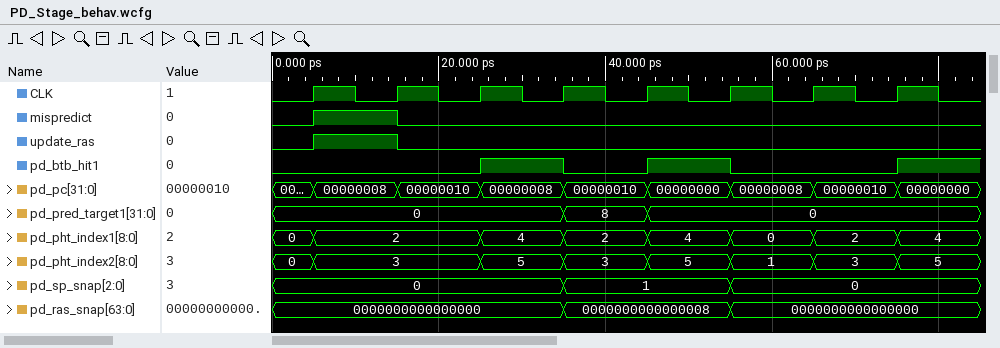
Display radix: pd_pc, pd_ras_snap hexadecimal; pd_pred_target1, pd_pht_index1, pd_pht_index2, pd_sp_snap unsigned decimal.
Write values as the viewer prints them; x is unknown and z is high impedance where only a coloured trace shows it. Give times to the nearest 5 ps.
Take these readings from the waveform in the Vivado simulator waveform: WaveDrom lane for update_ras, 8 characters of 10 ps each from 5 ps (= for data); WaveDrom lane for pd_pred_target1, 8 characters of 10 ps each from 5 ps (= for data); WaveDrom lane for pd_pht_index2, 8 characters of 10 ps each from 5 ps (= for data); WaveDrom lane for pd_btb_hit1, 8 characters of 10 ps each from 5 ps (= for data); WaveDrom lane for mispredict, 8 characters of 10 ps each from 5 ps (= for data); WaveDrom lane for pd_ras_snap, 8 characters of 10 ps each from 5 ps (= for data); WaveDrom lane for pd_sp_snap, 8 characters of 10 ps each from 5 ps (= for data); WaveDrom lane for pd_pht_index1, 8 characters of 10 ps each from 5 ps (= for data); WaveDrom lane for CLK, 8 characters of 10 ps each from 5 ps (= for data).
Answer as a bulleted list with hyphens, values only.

- {name: 'update_ras', wave: '10......'}
- {name: 'pd_pred_target1', wave: '=..==...', data: '0 8 0'}
- {name: 'pd_pht_index2', wave: '=.======', data: '3 5 3 5 1 3 5'}
- {name: 'pd_btb_hit1', wave: '0.1010.1'}
- {name: 'mispredict', wave: '10......'}
- {name: 'pd_ras_snap', wave: '=..=.=..', data: '0000000000000000 0000000000000008 0000000000000000'}
- {name: 'pd_sp_snap', wave: '=..=.=..', data: '0 1 0'}
- {name: 'pd_pht_index1', wave: '=.======', data: '2 4 2 4 0 2 4'}
- {name: 'CLK', wave: 'p.......'}
